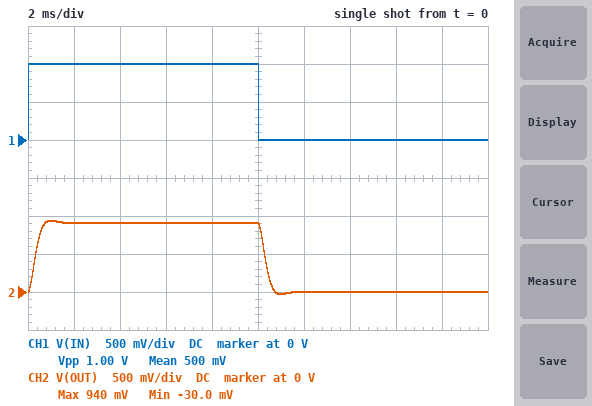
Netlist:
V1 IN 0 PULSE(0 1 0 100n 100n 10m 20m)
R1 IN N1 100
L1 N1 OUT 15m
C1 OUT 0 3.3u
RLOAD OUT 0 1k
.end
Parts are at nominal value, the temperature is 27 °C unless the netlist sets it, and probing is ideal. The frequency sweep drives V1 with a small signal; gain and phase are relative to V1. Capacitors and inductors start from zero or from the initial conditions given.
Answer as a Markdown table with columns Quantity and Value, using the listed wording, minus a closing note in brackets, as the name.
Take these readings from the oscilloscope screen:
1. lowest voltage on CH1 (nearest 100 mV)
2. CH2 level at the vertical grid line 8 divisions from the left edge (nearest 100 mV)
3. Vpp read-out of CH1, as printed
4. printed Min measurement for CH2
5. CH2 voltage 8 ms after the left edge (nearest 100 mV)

| Quantity | Value |
|---|---|
| lowest voltage on CH1 | 0 V |
| CH2 level at the vertical grid line 8 divisions from the left edge | 0 V |
| Vpp read-out of CH1, as printed | 1.00 V |
| printed Min measurement for CH2 | -30.0 mV |
| CH2 voltage 8 ms after the left edge | 900 mV |
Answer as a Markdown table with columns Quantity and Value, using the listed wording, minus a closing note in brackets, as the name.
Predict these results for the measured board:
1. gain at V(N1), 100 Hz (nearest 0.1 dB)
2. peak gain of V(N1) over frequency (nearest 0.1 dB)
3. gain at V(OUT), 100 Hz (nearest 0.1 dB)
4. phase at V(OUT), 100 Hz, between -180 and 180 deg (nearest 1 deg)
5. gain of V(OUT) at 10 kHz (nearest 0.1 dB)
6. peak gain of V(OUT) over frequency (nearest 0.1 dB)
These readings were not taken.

| Quantity | Value |
|---|---|
| gain at V(N1), 100 Hz | -1.0 dB |
| peak gain of V(N1) over frequency | 0 dB |
| gain at V(OUT), 100 Hz | -0.8 dB |
| phase at V(OUT), 100 Hz, between -180 and 180 deg | -11 deg |
| gain of V(OUT) at 10 kHz | -45.8 dB |
| peak gain of V(OUT) over frequency | -0.8 dB |
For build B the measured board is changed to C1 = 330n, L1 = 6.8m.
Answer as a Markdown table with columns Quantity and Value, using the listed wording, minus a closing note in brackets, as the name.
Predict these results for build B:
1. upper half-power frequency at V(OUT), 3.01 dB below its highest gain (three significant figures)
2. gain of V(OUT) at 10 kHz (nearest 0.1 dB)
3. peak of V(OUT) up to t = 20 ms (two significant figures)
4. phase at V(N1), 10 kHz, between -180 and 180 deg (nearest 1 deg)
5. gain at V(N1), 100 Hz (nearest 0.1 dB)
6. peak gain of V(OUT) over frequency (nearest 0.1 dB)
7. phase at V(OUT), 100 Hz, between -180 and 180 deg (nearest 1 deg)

| Quantity | Value |
|---|---|
| upper half-power frequency at V(OUT), 3.01 dB below its highest gain | 4.19 kHz |
| gain of V(OUT) at 10 kHz | -18.2 dB |
| peak of V(OUT) up to t = 20 ms | 1.1 V |
| phase at V(N1), 10 kHz, between -180 and 180 deg | 15 deg |
| gain at V(N1), 100 Hz | -0.8 dB |
| peak gain of V(OUT) over frequency | 1.9 dB |
| phase at V(OUT), 100 Hz, between -180 and 180 deg | -1 deg |
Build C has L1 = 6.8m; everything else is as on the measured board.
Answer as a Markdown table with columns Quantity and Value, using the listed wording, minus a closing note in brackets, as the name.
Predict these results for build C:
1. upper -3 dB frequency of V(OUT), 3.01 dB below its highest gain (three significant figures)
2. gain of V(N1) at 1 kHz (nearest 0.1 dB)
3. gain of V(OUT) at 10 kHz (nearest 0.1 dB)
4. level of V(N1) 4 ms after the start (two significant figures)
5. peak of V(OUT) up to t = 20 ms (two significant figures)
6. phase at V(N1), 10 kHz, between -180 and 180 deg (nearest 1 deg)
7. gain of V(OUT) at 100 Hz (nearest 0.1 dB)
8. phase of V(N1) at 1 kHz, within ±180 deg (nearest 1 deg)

| Quantity | Value |
|---|---|
| upper -3 dB frequency of V(OUT), 3.01 dB below its highest gain | 650 Hz |
| gain of V(N1) at 1 kHz | -24.8 dB |
| gain of V(OUT) at 10 kHz | -39.1 dB |
| level of V(N1) 4 ms after the start | 910 mV |
| peak of V(OUT) up to t = 20 ms | 910 mV |
| phase at V(N1), 10 kHz, between -180 and 180 deg | 13 deg |
| gain of V(OUT) at 100 Hz | -0.9 dB |
| phase of V(N1) at 1 kHz, within ±180 deg | -64 deg |
